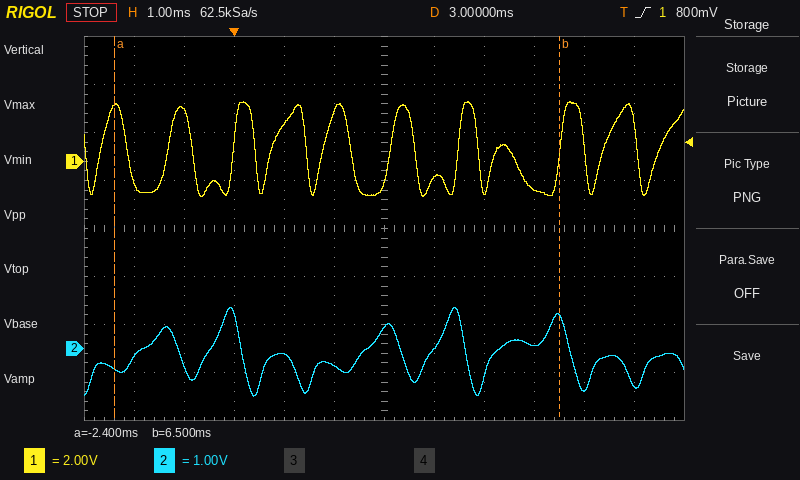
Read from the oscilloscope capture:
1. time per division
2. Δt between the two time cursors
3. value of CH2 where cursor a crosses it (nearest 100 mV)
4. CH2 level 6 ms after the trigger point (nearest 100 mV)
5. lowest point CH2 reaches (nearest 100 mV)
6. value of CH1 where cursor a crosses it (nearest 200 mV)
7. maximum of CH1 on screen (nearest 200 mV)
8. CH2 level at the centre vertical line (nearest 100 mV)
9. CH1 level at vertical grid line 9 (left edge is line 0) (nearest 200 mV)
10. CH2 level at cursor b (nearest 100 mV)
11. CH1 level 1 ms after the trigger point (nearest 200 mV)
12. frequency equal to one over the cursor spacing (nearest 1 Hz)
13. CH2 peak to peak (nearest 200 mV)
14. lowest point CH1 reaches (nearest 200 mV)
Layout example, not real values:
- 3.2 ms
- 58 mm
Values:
- 1 ms
- 8.9 ms
- -400 mV
- 100 mV
- -1.0 V
- 2.2 V
- 2.4 V
- 400 mV
- -1.2 V
- 600 mV
- 1.6 V
- 112 Hz
- 1.8 V
- -1.4 V
